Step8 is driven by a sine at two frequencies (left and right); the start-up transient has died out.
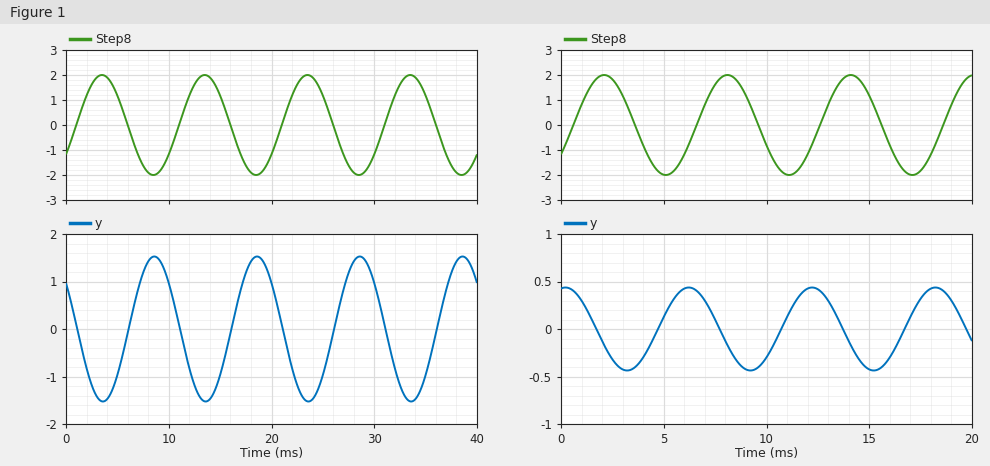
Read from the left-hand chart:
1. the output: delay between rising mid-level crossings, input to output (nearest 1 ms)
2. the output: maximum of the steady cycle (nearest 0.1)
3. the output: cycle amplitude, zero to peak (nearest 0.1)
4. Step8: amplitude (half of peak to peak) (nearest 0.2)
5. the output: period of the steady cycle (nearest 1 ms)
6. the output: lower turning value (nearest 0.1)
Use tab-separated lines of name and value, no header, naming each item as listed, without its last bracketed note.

the output: delay between rising mid-level crossings, input to output	5 ms
the output: maximum of the steady cycle	1.5
the output: cycle amplitude, zero to peak	1.5
Step8: amplitude (half of peak to peak)	2.0
the output: period of the steady cycle	10 ms
the output: lower turning value	-1.5
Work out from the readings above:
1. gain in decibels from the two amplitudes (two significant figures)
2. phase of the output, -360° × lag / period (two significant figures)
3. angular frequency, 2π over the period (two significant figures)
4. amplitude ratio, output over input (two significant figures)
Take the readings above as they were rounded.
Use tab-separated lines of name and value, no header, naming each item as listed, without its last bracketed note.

gain in decibels from the two amplitudes	-2.5 dB
phase of the output, -360° × lag / period	-180°
angular frequency, 2π over the period	0.63 rad/ms
amplitude ratio, output over input	0.75
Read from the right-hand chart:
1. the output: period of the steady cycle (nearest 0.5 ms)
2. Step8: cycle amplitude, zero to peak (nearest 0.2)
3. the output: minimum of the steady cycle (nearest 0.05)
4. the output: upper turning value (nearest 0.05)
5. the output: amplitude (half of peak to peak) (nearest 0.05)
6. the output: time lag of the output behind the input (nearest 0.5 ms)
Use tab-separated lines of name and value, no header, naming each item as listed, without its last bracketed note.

the output: period of the steady cycle	6.0 ms
Step8: cycle amplitude, zero to peak	2.0
the output: minimum of the steady cycle	-0.45
the output: upper turning value	0.45
the output: amplitude (half of peak to peak)	0.45
the output: time lag of the output behind the input	4.0 ms
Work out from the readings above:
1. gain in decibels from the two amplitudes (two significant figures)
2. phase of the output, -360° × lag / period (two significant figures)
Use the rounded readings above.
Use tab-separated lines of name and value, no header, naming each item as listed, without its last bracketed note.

gain in decibels from the two amplitudes	-13 dB
phase of the output, -360° × lag / period	-240°
